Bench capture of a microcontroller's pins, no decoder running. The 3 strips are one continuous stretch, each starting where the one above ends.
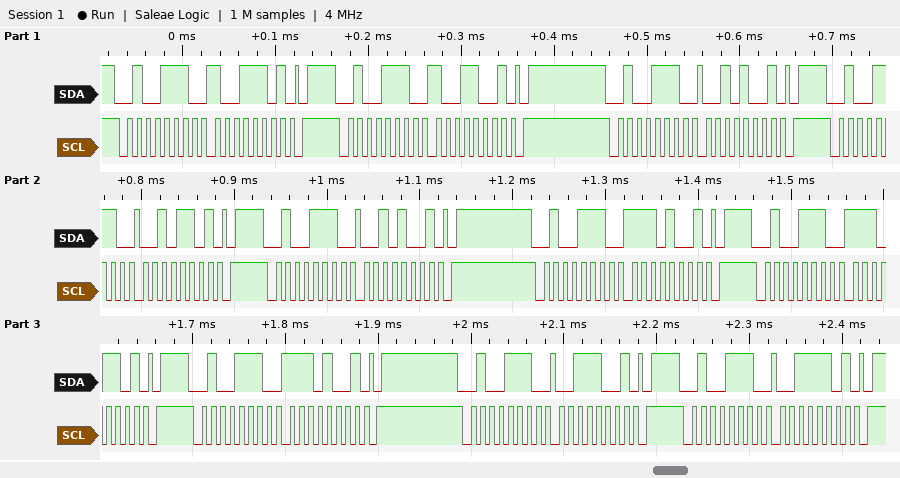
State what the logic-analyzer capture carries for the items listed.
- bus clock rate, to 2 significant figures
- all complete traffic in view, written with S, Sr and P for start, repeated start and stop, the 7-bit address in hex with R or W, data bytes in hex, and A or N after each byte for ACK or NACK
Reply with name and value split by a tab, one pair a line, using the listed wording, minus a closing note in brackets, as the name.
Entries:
bus clock rate, to 2 significant figures	100 kHz
all complete traffic in view, written with S, Sr and P for start, repeated start and stop, the 7-bit address in hex with R or W, data bytes in hex, and A or N after each byte for ACK or NACK	S 27W A 9D A P S 27W A 99 A P S 27W A 29 A P S 27W A 2D A P S 27W A 29 A P S 27W A E9 A P S 27W A ED A P S 27W A E9 A P S 27W A 39 A P S 27W A 3D A P
